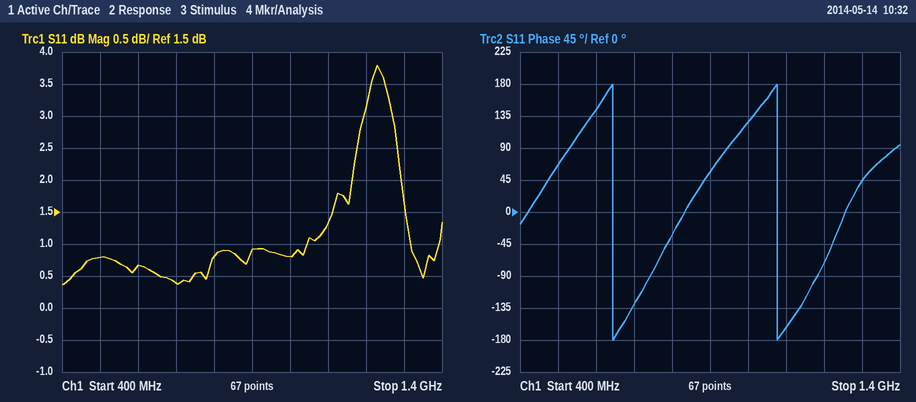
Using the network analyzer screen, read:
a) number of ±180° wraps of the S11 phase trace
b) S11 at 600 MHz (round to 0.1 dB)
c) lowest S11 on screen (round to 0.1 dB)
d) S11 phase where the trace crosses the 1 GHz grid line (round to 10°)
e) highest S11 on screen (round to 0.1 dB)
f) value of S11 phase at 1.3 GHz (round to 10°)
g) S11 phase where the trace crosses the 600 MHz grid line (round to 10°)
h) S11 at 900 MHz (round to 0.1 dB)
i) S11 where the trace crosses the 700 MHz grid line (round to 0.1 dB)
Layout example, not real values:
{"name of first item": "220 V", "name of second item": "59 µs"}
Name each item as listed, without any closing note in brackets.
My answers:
{"number of ±180° wraps of the S11 phase trace": "2", "S11 at 600 MHz": "0.7 dB", "lowest S11 on screen": "0.4 dB", "S11 phase where the trace crosses the 1 GHz grid line": "130°", "highest S11 on screen": "3.8 dB", "value of S11 phase at 1.3 GHz": "40°", "S11 phase where the trace crosses the 600 MHz grid line": "140°", "S11 at 900 MHz": "0.9 dB", "S11 where the trace crosses the 700 MHz grid line": "0.4 dB"}
